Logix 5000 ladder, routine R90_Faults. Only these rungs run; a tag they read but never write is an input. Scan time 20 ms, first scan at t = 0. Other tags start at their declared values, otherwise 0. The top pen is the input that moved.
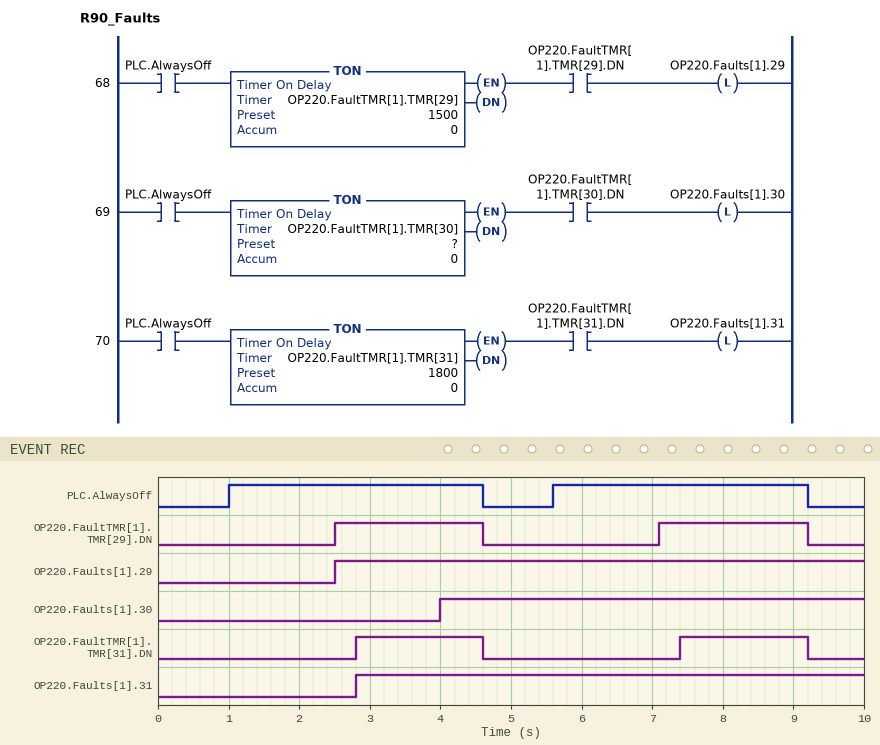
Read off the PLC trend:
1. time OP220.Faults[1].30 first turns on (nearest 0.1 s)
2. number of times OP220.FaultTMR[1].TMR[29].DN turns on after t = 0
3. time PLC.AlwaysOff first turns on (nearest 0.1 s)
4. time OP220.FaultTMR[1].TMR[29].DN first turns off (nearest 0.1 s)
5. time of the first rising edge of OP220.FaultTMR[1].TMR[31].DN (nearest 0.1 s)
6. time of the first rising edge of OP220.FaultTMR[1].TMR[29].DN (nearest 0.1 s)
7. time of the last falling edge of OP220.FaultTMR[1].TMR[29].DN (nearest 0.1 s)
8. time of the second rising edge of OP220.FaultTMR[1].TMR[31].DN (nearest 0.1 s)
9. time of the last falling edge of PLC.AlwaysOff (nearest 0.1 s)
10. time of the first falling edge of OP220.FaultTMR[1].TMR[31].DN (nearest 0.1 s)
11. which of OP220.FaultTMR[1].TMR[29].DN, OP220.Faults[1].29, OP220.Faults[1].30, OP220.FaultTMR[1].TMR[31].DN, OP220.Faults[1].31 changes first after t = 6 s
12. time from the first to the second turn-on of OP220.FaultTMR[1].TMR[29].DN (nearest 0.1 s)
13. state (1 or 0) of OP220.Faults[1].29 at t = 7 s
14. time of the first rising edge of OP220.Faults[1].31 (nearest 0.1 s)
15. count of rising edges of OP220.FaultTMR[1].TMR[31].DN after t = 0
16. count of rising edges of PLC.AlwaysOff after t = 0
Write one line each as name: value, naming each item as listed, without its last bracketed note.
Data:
time OP220.Faults[1].30 first turns on: 4.0 s
number of times OP220.FaultTMR[1].TMR[29].DN turns on after t = 0: 2
time PLC.AlwaysOff first turns on: 1.0 s
time OP220.FaultTMR[1].TMR[29].DN first turns off: 4.6 s
time of the first rising edge of OP220.FaultTMR[1].TMR[31].DN: 2.8 s
time of the first rising edge of OP220.FaultTMR[1].TMR[29].DN: 2.5 s
time of the last falling edge of OP220.FaultTMR[1].TMR[29].DN: 9.2 s
time of the second rising edge of OP220.FaultTMR[1].TMR[31].DN: 7.4 s
time of the last falling edge of PLC.AlwaysOff: 9.2 s
time of the first falling edge of OP220.FaultTMR[1].TMR[31].DN: 4.6 s
which of OP220.FaultTMR[1].TMR[29].DN, OP220.Faults[1].29, OP220.Faults[1].30, OP220.FaultTMR[1].TMR[31].DN, OP220.Faults[1].31 changes first after t = 6 s: OP220.FaultTMR[1].TMR[29].DN
time from the first to the second turn-on of OP220.FaultTMR[1].TMR[29].DN: 4.6 s
state (1 or 0) of OP220.Faults[1].29 at t = 7 s: 1
time of the first rising edge of OP220.Faults[1].31: 2.8 s
count of rising edges of OP220.FaultTMR[1].TMR[31].DN after t = 0: 2
count of rising edges of PLC.AlwaysOff after t = 0: 2
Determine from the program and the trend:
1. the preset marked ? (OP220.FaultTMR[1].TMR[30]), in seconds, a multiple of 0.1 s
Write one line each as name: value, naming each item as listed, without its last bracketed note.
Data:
the preset marked ? (OP220.FaultTMR[1].TMR[30]), in seconds, a multiple of 0.1 s: 3.0 s
